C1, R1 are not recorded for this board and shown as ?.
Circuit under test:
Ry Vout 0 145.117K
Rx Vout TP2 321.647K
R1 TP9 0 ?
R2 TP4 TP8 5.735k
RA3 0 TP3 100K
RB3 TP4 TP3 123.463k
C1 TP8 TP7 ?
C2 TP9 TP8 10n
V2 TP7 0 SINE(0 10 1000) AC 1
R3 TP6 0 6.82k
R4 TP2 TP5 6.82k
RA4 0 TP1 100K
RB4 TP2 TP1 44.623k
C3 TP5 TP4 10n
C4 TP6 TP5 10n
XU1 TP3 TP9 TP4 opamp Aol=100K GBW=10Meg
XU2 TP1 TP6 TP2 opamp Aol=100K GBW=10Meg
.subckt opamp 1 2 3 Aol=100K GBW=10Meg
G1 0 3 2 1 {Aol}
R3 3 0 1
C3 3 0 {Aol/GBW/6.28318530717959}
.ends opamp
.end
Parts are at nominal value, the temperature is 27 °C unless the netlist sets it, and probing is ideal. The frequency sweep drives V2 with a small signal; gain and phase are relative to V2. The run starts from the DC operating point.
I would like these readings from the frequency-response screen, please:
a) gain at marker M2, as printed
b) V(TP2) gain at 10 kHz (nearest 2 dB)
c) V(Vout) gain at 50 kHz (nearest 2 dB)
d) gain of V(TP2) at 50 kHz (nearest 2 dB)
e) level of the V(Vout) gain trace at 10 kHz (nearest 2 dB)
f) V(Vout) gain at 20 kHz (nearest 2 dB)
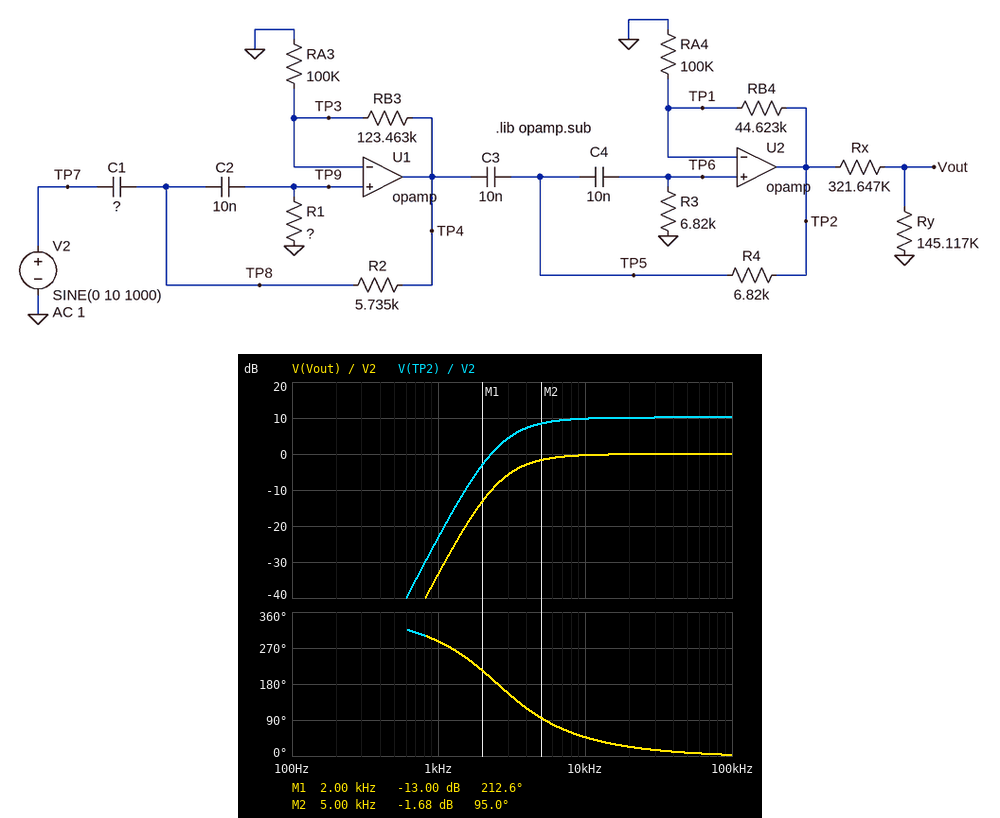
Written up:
-1.68 dB
10 dB
0 dB
10 dB
0 dB
0 dB
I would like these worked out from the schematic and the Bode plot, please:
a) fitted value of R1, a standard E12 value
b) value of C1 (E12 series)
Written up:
3.9 kΩ
15 nF
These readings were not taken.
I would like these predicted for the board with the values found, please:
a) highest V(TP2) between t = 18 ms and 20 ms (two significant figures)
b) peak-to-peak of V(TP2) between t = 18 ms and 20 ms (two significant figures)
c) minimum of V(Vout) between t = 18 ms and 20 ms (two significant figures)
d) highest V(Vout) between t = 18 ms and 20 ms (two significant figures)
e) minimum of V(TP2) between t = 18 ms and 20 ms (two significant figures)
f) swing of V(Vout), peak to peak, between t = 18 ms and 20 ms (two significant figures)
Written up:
710 mV
1.4 V
-220 mV
220 mV
-710 mV
440 mV
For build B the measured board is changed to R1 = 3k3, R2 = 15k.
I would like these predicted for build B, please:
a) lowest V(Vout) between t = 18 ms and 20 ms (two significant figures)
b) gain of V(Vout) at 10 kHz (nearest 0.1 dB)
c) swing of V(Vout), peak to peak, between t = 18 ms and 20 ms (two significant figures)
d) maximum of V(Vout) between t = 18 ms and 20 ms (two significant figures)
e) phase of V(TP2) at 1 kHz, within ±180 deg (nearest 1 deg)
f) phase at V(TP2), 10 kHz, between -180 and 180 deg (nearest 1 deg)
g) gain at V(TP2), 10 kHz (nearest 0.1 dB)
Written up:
-230 mV
-1.7 dB
460 mV
230 mV
-111 deg
57 deg
8.5 dB
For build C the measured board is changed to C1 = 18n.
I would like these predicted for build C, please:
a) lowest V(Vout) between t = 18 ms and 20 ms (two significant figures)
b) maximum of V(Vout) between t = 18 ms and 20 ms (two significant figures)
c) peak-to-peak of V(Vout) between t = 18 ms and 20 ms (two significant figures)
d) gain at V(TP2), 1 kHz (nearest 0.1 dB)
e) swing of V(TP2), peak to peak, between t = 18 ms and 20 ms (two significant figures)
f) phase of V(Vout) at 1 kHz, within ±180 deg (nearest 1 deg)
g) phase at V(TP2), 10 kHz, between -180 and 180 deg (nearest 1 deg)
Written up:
-250 mV
250 mV
510 mV
-21.8 dB
1.6 V
-79 deg
46 deg
